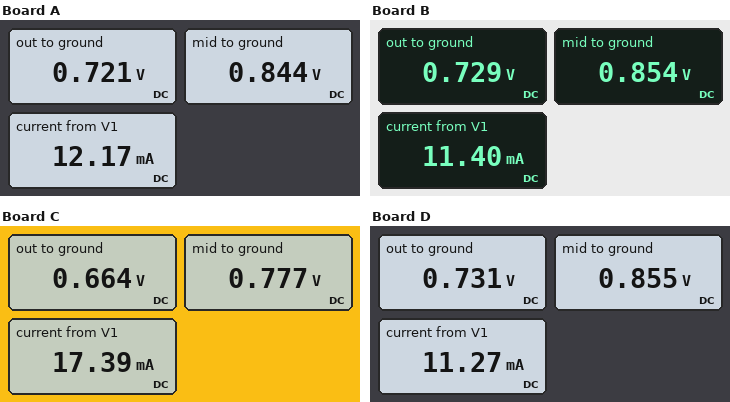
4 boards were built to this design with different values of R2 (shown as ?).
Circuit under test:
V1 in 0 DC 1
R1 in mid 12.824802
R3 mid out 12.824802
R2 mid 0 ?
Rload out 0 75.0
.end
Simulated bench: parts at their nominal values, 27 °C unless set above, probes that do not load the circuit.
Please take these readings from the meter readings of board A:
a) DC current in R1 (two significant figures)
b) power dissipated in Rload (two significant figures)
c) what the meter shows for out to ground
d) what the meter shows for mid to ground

12 mA
6.9 mW
0.721 V
0.844 V
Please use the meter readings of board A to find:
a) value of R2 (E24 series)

330 Ω
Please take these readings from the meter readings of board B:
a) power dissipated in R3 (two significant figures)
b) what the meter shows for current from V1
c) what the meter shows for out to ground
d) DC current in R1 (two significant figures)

1.2 mW
11.40 mA
0.729 V
11 mA
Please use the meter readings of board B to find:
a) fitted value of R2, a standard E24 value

510 Ω
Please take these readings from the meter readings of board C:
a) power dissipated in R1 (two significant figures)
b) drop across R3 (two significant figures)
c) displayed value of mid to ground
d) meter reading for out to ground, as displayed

3.9 mW
110 mV
0.777 V
0.664 V
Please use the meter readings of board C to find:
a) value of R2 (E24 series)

91 Ω
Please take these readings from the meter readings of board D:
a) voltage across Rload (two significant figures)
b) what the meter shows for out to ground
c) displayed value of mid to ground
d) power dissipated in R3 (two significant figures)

730 mV
0.731 V
0.855 V
1.2 mW
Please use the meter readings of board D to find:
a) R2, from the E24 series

560 Ω
